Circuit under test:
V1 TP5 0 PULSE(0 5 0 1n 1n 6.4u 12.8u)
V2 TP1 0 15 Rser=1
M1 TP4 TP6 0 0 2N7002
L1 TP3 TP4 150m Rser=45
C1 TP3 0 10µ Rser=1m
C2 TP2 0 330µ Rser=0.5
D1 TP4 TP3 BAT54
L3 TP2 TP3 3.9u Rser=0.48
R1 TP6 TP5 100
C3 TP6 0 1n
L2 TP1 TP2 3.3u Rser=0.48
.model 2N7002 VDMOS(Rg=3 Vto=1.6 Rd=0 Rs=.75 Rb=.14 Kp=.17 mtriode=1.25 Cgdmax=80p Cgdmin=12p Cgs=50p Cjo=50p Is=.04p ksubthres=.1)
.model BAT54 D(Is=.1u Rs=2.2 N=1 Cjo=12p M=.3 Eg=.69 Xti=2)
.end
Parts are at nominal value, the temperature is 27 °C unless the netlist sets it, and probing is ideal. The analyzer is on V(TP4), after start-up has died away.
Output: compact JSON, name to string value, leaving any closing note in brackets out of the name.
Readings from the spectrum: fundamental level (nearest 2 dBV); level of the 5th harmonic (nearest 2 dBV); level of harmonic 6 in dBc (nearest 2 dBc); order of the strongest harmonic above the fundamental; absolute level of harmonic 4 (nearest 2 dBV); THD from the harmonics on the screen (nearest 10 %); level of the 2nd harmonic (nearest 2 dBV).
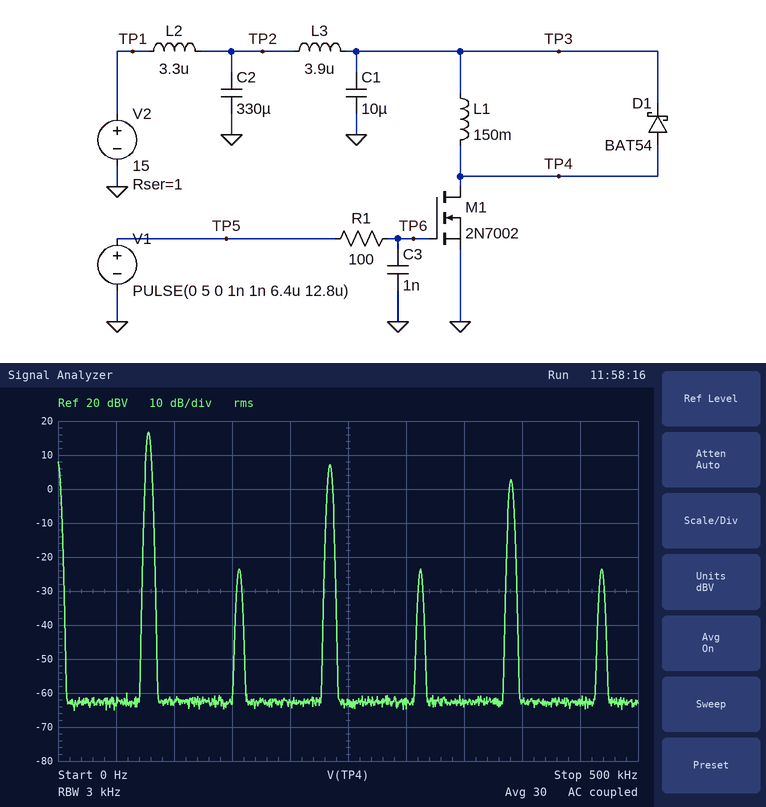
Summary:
{"fundamental level": "16 dBV", "level of the 5th harmonic": "2 dBV", "level of harmonic 6 in dBc": "-40 dBc", "order of the strongest harmonic above the fundamental": "3", "absolute level of harmonic 4": "-24 dBV", "THD from the harmonics on the screen": "40 %", "level of the 2nd harmonic": "-24 dBV"}
